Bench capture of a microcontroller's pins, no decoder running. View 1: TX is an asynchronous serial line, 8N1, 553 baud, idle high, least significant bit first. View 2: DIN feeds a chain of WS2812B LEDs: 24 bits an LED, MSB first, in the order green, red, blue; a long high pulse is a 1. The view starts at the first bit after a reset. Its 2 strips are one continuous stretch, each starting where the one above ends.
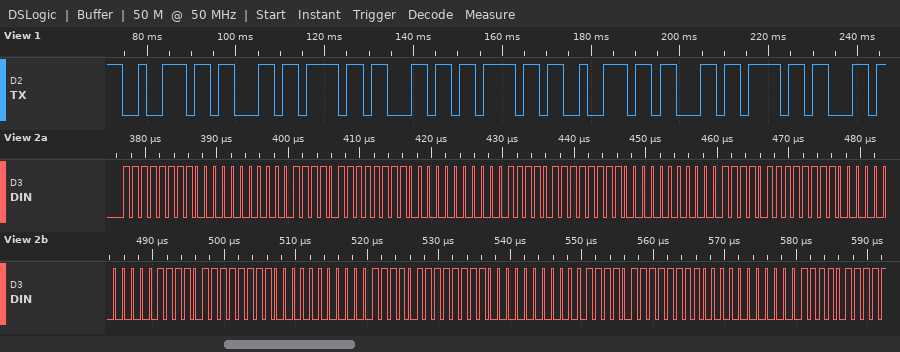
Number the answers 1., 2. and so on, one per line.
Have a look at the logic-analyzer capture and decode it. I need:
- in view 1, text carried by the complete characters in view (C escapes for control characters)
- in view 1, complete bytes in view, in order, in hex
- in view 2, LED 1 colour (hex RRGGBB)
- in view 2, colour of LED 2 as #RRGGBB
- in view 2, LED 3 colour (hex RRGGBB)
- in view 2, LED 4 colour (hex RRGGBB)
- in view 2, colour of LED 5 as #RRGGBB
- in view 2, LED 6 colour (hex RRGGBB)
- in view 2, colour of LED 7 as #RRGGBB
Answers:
1. "rcolorco"
2. 0x72 0x63 0x6F 0x6C 0x6F 0x72 0x63 0x6F
3. #00FF1E
4. #00FF1E
5. #00FF1E
6. #00FF1E
7. #00FF1E
8. #00FF1E
9. #00FF1E
